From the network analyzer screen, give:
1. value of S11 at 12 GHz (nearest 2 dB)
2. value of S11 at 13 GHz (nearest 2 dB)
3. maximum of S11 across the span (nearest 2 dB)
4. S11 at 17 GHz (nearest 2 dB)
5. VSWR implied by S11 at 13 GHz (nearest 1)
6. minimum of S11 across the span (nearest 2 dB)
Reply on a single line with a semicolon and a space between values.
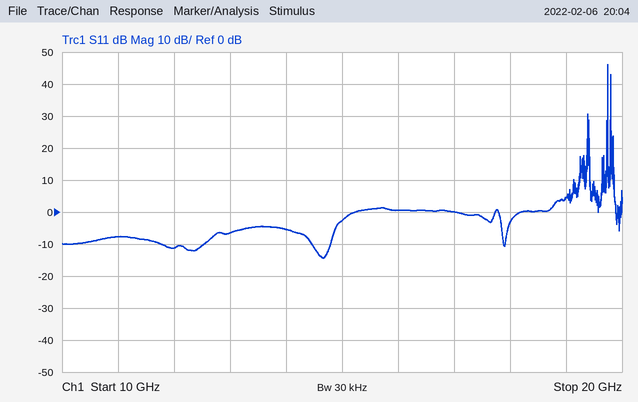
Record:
-12 dB; -6 dB; 46 dB; 0 dB; 3; -14 dB
